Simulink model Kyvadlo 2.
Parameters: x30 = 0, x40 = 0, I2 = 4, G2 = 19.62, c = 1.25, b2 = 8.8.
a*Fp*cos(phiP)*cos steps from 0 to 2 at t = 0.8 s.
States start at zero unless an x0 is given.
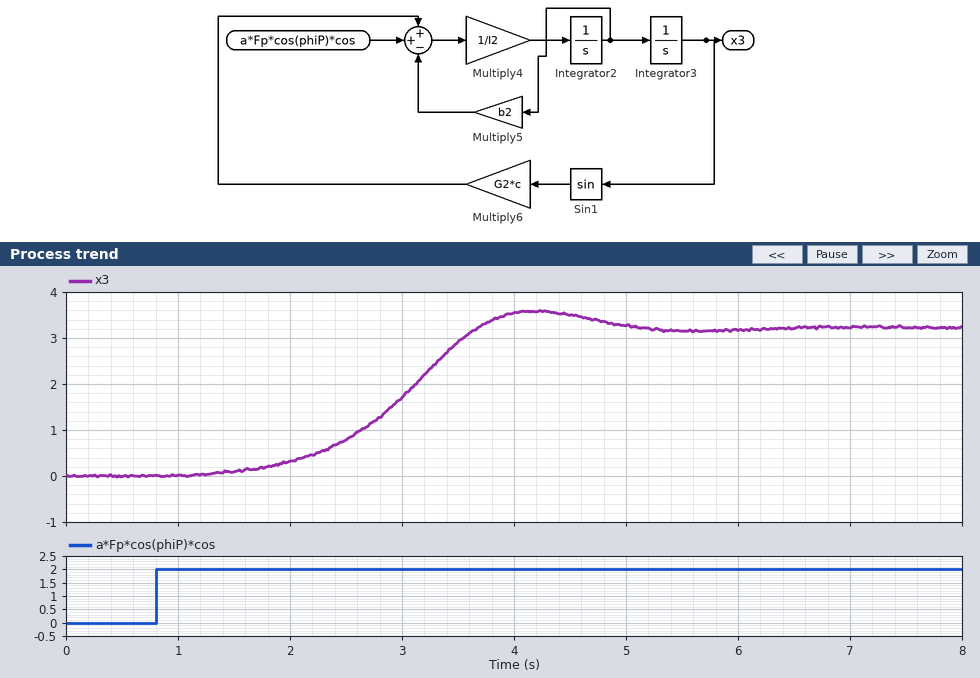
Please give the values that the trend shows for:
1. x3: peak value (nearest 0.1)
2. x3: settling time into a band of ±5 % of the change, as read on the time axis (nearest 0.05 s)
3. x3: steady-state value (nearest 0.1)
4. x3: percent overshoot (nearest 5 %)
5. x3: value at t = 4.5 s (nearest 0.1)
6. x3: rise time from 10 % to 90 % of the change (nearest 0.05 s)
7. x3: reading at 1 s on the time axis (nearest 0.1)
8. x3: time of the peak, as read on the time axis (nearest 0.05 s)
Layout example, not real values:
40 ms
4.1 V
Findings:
3.6
4.75 s
3.2
10 %
3.5
1.50 s
0.0
4.20 s
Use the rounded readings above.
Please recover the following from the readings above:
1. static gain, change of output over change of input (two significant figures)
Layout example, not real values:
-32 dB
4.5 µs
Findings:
1.6
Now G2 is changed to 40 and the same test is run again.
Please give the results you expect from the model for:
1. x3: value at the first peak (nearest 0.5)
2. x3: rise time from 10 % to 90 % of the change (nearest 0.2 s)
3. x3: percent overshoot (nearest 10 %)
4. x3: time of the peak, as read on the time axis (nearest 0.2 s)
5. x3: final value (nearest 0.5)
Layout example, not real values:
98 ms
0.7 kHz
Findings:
4.0
1.0 s
20 %
3.2 s
3.0
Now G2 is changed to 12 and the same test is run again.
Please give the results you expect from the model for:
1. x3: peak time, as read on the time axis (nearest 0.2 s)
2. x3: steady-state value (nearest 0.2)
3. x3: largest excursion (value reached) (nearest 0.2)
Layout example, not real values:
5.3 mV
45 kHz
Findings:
5.2 s
3.2
3.4
